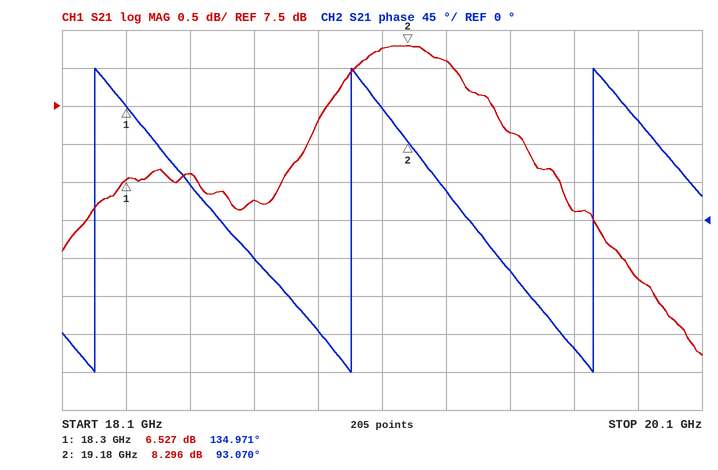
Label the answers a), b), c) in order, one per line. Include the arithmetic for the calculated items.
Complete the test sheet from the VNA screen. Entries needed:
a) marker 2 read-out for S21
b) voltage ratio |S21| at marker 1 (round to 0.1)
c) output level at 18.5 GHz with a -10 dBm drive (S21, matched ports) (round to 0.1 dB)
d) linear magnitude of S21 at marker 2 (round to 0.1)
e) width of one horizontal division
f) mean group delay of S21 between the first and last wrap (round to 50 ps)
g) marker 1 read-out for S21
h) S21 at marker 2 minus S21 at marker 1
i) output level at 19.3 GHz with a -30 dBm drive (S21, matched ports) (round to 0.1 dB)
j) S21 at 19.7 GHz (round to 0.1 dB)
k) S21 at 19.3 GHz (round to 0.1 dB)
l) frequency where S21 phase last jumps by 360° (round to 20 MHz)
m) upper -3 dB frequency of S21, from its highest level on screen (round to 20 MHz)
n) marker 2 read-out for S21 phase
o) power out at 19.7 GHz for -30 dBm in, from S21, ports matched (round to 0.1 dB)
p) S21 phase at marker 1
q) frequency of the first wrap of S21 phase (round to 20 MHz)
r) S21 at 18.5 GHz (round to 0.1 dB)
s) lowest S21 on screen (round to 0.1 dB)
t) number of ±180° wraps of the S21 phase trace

a) 8.296 dB
b) 10^(6.527/20) ≈ 2.1
c) -10 dBm + (6.6 dB) = -3.4 dBm
d) 10^(8.296/20) ≈ 2.6
e) 200 MHz
f) 2 cycles / (19.76 GHz − 18.20 GHz) ≈ 1.28 ns, so 1.30 ns to the nearest 50 ps
g) 6.527 dB
h) 8.296 − (6.527) = 1.769 dB
i) -30 dBm + (8.1 dB) = -21.9 dBm
j) 6.1 dB
k) 8.1 dB
l) 19.76 GHz
m) 19.88 GHz
n) 93.070°
o) -30 dBm + (6.1 dB) = -23.9 dBm
p) 134.971°
q) 18.20 GHz
r) 6.6 dB
s) 4.2 dB
t) 3
